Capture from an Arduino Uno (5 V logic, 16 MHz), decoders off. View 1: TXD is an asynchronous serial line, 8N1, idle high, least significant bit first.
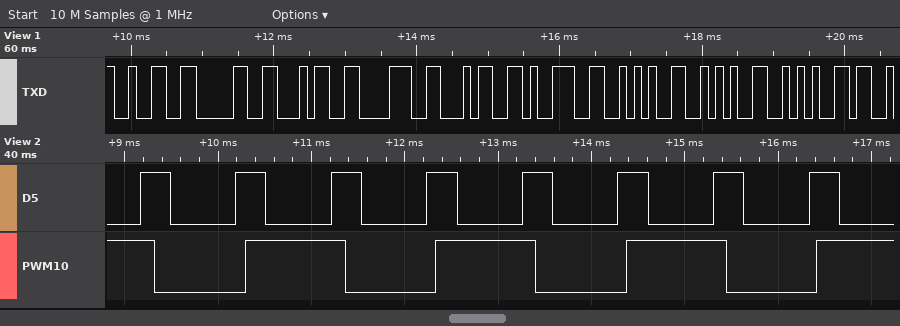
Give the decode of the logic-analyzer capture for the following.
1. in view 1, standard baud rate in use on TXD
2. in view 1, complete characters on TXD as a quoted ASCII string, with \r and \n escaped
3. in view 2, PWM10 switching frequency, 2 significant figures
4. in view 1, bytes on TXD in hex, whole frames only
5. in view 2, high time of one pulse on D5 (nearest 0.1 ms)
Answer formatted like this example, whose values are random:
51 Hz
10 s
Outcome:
9600 baud
"204849***"
490 Hz
0x32 0x30 0x34 0x38 0x34 0x39 0x2A 0x2A 0x2A
0.3 ms
